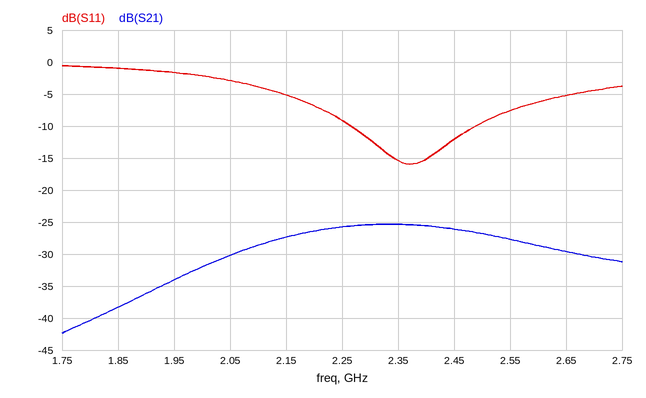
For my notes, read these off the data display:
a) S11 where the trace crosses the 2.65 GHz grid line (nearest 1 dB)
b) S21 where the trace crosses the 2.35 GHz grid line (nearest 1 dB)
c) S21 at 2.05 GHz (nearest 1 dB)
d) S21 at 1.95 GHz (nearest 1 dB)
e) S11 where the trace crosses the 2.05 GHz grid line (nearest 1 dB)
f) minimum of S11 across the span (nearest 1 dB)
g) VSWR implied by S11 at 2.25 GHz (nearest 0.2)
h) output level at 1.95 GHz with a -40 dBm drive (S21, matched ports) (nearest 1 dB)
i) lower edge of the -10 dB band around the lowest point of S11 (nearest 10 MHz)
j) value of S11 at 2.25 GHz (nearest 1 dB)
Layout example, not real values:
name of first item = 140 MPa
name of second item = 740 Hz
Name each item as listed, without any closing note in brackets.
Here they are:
S11 where the trace crosses the 2.65 GHz grid line = -5 dB
S21 where the trace crosses the 2.35 GHz grid line = -25 dB
S21 at 2.05 GHz = -30 dB
S21 at 1.95 GHz = -34 dB
S11 where the trace crosses the 2.05 GHz grid line = -3 dB
minimum of S11 across the span = -16 dB
VSWR implied by S11 at 2.25 GHz = 2.0
output level at 1.95 GHz with a -40 dBm drive (S21, matched ports) = -74 dBm
lower edge of the -10 dB band around the lowest point of S11 = 2.27 GHz
value of S11 at 2.25 GHz = -9 dB
